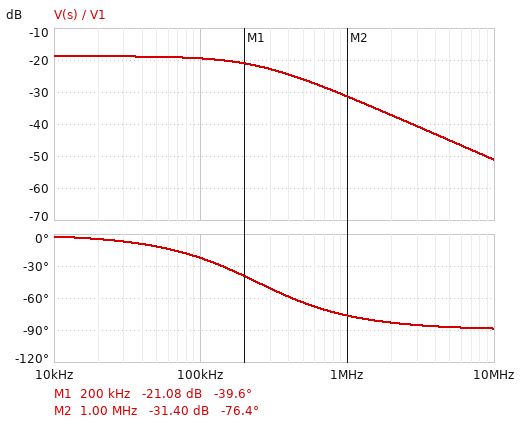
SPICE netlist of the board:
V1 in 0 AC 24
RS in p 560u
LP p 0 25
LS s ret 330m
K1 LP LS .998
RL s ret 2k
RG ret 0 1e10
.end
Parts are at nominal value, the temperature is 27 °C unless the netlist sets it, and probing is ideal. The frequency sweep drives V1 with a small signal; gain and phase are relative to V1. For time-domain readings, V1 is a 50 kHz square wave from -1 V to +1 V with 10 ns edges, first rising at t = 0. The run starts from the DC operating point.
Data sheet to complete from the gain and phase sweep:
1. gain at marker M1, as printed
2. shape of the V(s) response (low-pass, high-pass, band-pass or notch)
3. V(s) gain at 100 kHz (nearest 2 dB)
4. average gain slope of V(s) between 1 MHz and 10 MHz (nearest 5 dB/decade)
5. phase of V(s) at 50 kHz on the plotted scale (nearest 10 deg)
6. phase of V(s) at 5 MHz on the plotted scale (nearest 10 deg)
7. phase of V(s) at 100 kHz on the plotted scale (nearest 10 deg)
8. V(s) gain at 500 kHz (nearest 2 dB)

-21.08 dB
low-pass
-20 dB
-20 dB/decade
-10 deg
-90 deg
-20 deg
-26 dB
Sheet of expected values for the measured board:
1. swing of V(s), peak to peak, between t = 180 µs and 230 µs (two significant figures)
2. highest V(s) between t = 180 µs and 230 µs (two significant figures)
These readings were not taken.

230 mV
230 mV
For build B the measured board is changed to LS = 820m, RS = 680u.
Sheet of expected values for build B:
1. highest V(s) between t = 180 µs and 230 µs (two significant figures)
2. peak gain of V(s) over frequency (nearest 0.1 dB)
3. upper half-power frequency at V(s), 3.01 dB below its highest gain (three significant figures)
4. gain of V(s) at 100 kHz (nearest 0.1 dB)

360 mV
-14.9 dB
97.1 kHz
-18.0 dB
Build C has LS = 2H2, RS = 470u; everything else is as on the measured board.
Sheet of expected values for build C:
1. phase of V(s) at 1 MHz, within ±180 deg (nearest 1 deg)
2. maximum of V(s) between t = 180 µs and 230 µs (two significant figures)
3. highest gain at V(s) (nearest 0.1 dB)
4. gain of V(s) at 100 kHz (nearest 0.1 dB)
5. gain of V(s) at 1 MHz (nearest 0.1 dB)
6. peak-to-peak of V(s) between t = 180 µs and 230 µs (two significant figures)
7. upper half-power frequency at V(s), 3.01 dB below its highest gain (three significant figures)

-88 deg
540 mV
-10.6 dB
-19.9 dB
-39.4 dB
480 mV
36.2 kHz
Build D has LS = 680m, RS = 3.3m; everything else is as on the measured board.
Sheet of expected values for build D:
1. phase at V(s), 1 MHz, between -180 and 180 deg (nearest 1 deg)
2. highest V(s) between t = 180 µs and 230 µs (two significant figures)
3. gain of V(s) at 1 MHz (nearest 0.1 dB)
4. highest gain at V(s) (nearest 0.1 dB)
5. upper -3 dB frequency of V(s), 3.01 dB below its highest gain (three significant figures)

-83 deg
330 mV
-34.4 dB
-15.7 dB
117 kHz
